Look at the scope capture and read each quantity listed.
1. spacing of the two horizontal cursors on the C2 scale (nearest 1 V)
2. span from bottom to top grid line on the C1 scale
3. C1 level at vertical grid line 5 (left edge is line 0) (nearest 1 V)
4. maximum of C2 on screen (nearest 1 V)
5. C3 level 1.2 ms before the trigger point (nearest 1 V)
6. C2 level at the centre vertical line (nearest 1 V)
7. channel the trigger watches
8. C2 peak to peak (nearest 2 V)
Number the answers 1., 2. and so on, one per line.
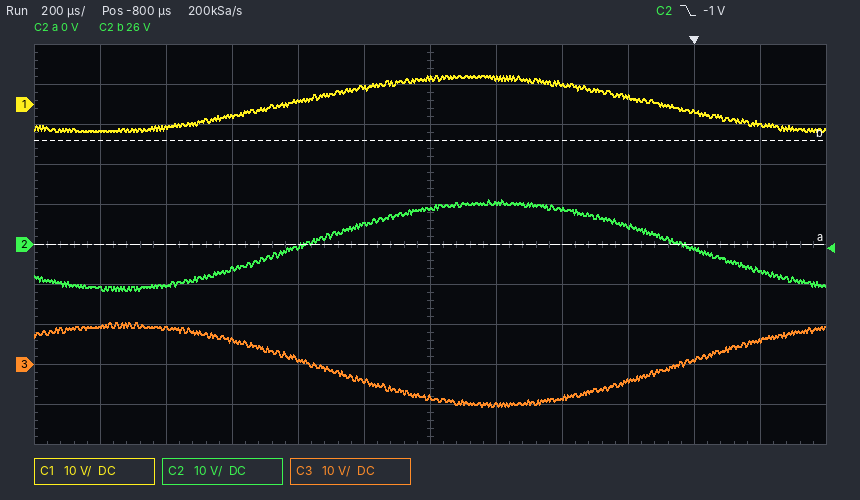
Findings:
1. 26 V
2. 100 V
3. 4 V
4. 11 V
5. 1 V
6. 9 V
7. C2
8. 22 V
